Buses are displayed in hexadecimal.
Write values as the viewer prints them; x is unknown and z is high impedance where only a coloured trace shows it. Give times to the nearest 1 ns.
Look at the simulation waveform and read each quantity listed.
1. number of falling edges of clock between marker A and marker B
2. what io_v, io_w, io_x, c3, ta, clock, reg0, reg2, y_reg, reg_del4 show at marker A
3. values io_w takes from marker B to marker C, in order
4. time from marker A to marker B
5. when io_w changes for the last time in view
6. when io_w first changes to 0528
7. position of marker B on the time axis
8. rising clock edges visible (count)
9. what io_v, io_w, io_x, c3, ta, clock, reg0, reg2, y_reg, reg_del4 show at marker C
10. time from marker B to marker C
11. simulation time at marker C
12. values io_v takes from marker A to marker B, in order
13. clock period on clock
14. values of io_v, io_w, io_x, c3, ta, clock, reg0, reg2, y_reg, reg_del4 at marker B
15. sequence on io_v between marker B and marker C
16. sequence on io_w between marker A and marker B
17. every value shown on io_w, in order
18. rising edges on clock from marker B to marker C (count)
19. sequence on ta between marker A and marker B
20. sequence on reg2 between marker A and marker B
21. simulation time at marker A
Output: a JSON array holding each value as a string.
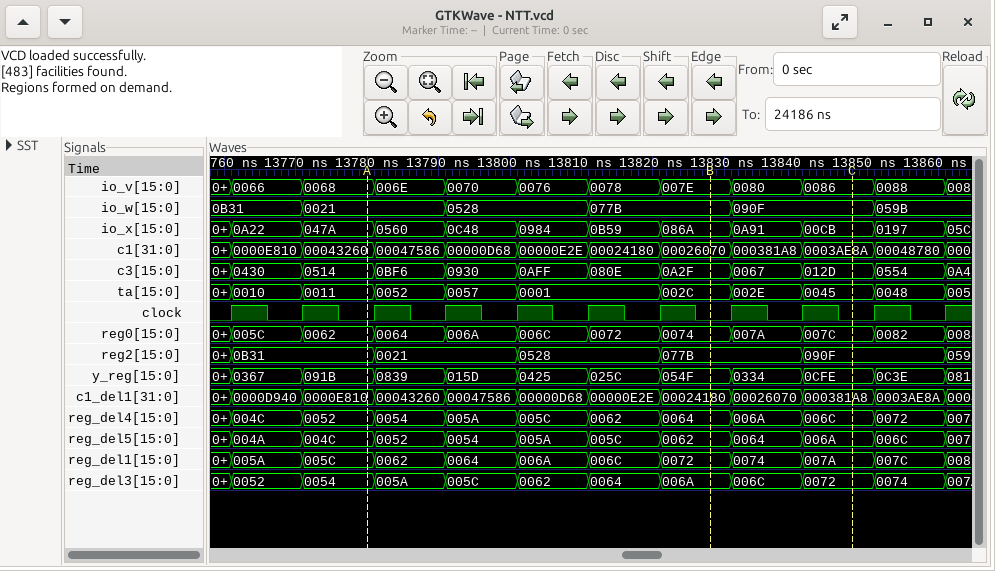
["5", "io_v=0068, io_w=0021, io_x=047A, c3=0514, ta=0011, clock=0, reg0=0062, reg2=0B31, y_reg=091B, reg_del4=0052", "077B, 090F", "48 ns", "13851 ns", "13791 ns", "13828 ns", "11", "io_v=0086, io_w=090F, io_x=00CB, c3=012D, ta=0045, clock=0, reg0=007C, reg2=090F, y_reg=0CFE, reg_del4=006C", "20 ns", "13848 ns", "0068, 006E, 0070, 0076, 0078, 007E", "10 ns", "io_v=007E, io_w=077B, io_x=086A, c3=0A2F, ta=002C, clock=0, reg0=0074, reg2=077B, y_reg=054F, reg_del4=0064", "007E, 0080, 0086", "0021, 0528, 077B", "0B31, 0021, 0528, 077B, 090F, 059B", "2", "0011, 0052, 0057, 0001, 002C", "0B31, 0021, 0528, 077B", "13780 ns"]
